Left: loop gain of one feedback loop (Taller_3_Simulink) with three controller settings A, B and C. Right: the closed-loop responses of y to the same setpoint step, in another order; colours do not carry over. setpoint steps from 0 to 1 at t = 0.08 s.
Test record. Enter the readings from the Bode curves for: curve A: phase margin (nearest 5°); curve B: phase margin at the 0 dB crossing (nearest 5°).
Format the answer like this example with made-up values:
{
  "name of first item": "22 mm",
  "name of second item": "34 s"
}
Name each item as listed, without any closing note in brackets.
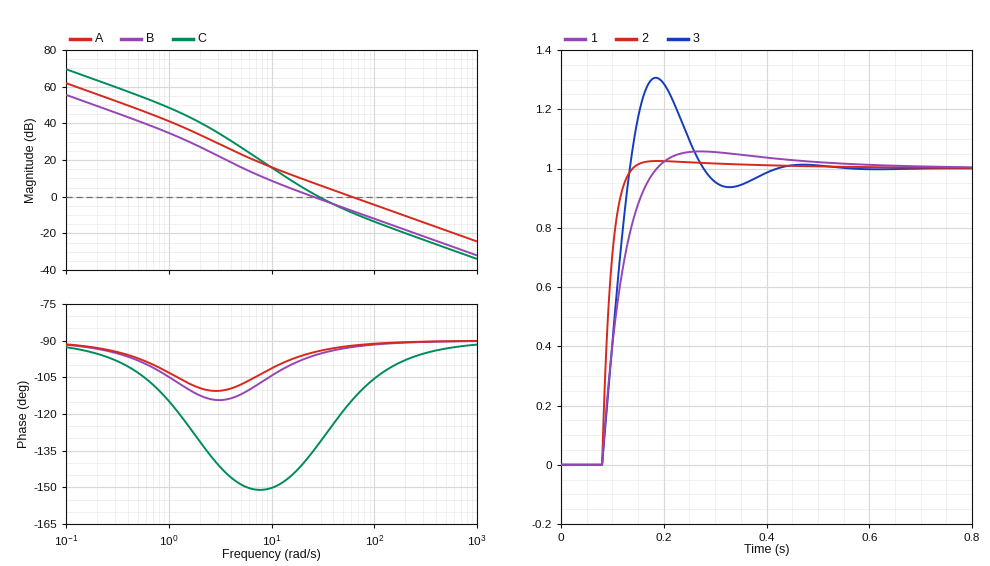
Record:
{
  "curve A: phase margin": "90°",
  "curve B: phase margin at the 0 dB crossing": "85°"
}
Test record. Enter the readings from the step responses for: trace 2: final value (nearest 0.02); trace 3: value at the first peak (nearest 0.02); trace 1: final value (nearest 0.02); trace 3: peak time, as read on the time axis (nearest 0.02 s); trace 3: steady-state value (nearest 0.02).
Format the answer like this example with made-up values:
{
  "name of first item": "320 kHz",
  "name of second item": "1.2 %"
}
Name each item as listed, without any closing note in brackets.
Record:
{
  "trace 2: final value": "1.00",
  "trace 3: value at the first peak": "1.30",
  "trace 1: final value": "1.00",
  "trace 3: peak time, as read on the time axis": "0.18 s",
  "trace 3: steady-state value": "1.00"
}
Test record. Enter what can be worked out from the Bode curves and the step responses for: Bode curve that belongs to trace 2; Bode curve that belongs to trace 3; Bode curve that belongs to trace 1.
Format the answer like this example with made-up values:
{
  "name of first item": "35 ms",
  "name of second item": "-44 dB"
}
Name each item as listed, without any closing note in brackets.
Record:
{
  "Bode curve that belongs to trace 2": "A",
  "Bode curve that belongs to trace 3": "C",
  "Bode curve that belongs to trace 1": "B"
}
